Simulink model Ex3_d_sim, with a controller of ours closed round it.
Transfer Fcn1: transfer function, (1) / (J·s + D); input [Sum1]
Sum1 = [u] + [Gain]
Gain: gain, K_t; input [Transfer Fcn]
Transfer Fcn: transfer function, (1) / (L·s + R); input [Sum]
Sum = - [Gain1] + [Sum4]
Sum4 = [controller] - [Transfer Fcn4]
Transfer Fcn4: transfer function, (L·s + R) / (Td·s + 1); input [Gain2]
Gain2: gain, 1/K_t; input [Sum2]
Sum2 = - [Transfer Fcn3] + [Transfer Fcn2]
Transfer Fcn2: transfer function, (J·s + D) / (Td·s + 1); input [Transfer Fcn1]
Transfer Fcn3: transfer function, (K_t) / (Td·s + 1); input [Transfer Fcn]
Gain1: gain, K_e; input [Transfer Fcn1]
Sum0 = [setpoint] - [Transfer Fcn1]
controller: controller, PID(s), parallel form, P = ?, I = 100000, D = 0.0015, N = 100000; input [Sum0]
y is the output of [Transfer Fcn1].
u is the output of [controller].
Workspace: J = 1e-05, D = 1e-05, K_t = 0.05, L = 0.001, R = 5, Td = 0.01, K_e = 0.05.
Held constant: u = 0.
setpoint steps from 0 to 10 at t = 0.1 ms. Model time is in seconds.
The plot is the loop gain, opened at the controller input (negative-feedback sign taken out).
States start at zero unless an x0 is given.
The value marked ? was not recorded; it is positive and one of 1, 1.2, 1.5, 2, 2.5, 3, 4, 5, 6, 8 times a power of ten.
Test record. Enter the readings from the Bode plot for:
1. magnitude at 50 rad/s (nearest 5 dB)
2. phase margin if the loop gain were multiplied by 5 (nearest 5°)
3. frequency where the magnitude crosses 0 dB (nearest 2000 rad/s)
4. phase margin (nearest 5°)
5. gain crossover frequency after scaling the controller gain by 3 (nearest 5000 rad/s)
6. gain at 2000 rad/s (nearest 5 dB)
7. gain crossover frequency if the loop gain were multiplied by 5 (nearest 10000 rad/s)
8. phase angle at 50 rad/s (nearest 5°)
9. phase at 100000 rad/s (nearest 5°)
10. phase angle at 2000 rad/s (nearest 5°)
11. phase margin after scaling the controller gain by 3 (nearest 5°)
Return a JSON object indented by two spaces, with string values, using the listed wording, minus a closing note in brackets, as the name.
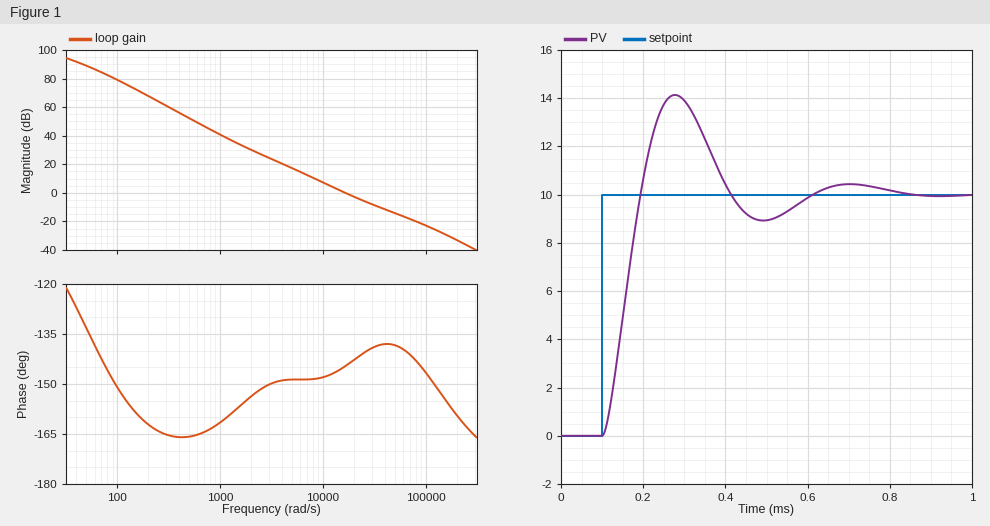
{
  "magnitude at 50 rad/s": "90 dB",
  "phase margin if the loop gain were multiplied by 5": "40°",
  "frequency where the magnitude crosses 0 dB": "16000 rad/s",
  "phase margin": "35°",
  "gain crossover frequency after scaling the controller gain by 3": "35000 rad/s",
  "gain at 2000 rad/s": "30 dB",
  "gain crossover frequency if the loop gain were multiplied by 5": "50000 rad/s",
  "phase angle at 50 rad/s": "-135°",
  "phase at 100000 rad/s": "-145°",
  "phase angle at 2000 rad/s": "-155°",
  "phase margin after scaling the controller gain by 3": "40°"
}
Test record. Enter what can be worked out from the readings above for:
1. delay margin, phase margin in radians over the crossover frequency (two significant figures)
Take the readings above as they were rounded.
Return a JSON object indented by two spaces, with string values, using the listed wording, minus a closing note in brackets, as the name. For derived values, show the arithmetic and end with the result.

{
  "delay margin, phase margin in radians over the crossover frequency": "35 × π / 180 / 16000 = 0.000038 s"
}
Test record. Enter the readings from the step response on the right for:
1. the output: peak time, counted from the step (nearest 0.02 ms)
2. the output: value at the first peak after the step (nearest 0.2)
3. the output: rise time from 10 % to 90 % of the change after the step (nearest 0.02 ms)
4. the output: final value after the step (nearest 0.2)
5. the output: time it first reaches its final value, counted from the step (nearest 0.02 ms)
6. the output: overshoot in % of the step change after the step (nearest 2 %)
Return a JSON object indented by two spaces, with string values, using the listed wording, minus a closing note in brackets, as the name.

{
  "the output: peak time, counted from the step": "0.18 ms",
  "the output: value at the first peak after the step": "14.2",
  "the output: rise time from 10 % to 90 % of the change after the step": "0.06 ms",
  "the output: final value after the step": "10.0",
  "the output: time it first reaches its final value, counted from the step": "0.10 ms",
  "the output: overshoot in % of the step change after the step": "42 %"
}
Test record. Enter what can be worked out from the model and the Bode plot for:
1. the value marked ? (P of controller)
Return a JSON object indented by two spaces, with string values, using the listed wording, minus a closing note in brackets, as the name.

{
  "the value marked ?": "50"
}
